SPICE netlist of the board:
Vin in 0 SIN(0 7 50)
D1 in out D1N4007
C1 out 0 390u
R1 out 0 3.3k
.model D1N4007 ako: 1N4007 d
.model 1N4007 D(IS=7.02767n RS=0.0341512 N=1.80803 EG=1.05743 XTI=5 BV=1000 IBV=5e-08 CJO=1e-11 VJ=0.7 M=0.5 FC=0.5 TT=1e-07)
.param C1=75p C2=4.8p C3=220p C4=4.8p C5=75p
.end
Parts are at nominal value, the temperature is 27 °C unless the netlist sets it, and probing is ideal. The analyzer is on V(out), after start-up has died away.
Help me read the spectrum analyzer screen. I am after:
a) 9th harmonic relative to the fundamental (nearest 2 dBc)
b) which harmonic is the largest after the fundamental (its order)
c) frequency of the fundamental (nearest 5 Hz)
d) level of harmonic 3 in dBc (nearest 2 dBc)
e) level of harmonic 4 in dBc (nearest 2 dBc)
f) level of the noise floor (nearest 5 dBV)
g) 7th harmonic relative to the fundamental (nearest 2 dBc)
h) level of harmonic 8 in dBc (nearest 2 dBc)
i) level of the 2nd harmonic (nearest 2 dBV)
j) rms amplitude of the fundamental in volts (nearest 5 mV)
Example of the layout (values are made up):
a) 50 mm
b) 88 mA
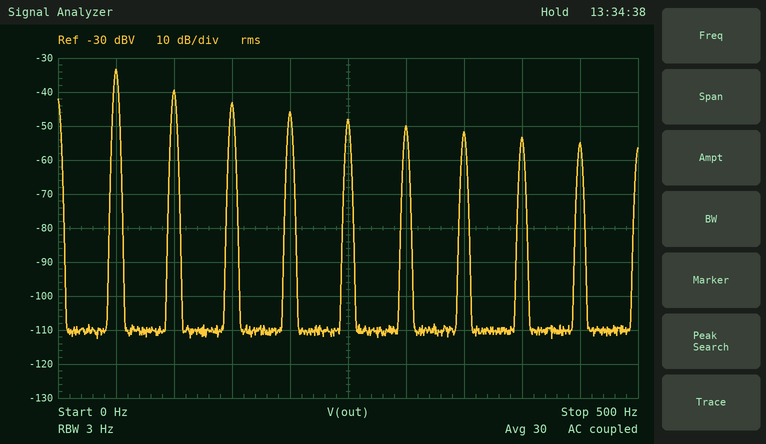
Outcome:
a) -22 dBc
b) 2
c) 50 Hz
d) -10 dBc
e) -12 dBc
f) -110 dBV
g) -18 dBc
h) -20 dBc
i) -40 dBV
j) 20 mV
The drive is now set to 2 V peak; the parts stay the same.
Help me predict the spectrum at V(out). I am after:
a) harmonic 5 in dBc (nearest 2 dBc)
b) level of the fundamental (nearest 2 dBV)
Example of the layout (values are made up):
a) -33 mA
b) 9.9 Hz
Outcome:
a) -16 dBc
b) -46 dBV
